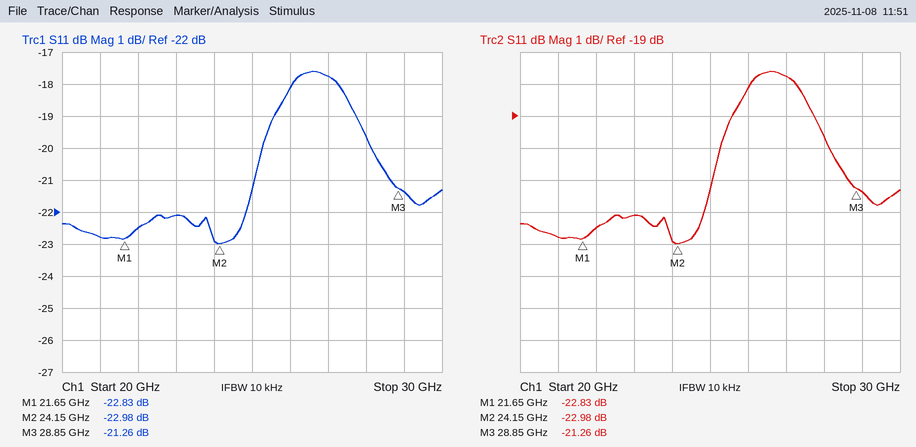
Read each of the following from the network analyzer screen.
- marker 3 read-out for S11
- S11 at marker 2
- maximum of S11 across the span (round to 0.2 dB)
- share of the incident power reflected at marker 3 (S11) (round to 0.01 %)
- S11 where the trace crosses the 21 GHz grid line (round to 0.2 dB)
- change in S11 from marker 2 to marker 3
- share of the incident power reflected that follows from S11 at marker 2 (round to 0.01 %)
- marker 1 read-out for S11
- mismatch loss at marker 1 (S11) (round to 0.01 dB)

-21.26 dB
-22.98 dB
-17.6 dB
0.75 %
-22.8 dB
1.72 dB
0.50 %
-22.83 dB
0.02 dB
